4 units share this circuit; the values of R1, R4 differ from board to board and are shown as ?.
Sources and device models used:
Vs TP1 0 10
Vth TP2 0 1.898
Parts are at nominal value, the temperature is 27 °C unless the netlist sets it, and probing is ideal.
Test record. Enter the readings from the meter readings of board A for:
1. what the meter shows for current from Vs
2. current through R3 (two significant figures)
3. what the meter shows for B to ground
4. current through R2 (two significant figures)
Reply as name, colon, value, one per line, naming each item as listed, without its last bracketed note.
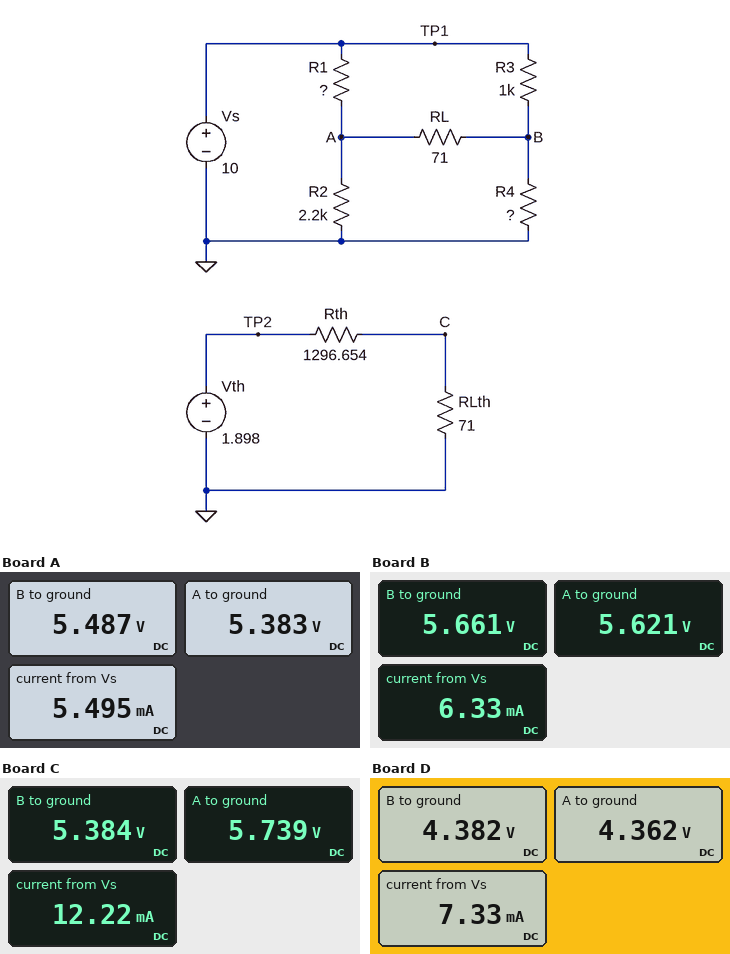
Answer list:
what the meter shows for current from Vs: 5.495 mA
current through R3: 4.5 mA
what the meter shows for B to ground: 5.487 V
current through R2: 2.4 mA
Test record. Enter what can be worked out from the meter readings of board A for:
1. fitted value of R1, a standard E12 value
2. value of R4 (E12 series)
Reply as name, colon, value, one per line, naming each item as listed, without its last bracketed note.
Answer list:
fitted value of R1, a standard E12 value: 4.7 kΩ
value of R4: 1.8 kΩ
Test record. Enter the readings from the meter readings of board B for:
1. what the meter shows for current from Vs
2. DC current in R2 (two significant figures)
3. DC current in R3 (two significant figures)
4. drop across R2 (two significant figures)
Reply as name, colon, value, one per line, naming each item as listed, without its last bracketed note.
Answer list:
what the meter shows for current from Vs: 6.33 mA
DC current in R2: 2.6 mA
DC current in R3: 4.3 mA
drop across R2: 5.6 V
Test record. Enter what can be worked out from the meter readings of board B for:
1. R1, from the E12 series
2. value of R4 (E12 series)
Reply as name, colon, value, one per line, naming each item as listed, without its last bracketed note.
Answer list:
R1, from the E12 series: 2.2 kΩ
value of R4: 1.5 kΩ
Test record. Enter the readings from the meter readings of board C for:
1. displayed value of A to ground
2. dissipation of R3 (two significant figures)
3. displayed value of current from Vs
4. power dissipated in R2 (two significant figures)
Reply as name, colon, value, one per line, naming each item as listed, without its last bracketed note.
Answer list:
displayed value of A to ground: 5.739 V
dissipation of R3: 21 mW
displayed value of current from Vs: 12.22 mA
power dissipated in R2: 15 mW
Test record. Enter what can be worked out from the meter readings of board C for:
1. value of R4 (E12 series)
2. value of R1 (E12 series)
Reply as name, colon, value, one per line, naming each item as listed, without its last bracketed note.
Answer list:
value of R4: 560 Ω
value of R1: 560 Ω
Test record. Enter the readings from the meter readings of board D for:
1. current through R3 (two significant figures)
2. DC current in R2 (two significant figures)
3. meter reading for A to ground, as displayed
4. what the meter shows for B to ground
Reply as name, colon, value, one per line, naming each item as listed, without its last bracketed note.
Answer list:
current through R3: 5.6 mA
DC current in R2: 2.0 mA
meter reading for A to ground, as displayed: 4.362 V
what the meter shows for B to ground: 4.382 V
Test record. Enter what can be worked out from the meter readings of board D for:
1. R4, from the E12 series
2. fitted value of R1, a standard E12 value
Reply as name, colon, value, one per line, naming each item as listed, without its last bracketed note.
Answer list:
R4, from the E12 series: 820 Ω
fitted value of R1, a standard E12 value: 3.3 kΩ
